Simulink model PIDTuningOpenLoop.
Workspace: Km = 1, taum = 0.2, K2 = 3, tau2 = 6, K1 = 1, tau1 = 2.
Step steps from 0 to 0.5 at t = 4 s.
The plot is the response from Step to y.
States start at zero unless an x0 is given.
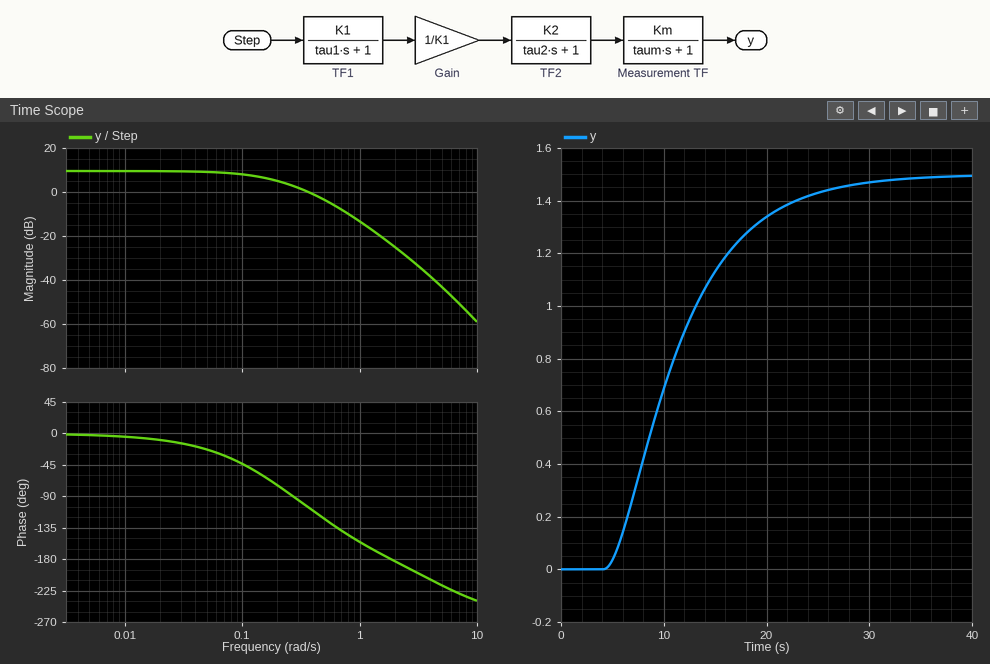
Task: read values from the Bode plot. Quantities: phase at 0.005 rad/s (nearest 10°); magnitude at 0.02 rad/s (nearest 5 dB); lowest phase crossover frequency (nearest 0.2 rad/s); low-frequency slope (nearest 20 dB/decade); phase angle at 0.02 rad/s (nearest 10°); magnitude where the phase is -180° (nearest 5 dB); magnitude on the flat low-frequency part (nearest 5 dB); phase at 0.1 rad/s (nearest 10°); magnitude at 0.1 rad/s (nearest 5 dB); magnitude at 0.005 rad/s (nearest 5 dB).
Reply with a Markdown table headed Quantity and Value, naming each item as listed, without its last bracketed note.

| Quantity | Value |
|---|---|
| phase at 0.005 rad/s | 0° |
| magnitude at 0.02 rad/s | 10 dB |
| lowest phase crossover frequency | 1.8 rad/s |
| low-frequency slope | 0 dB/decade |
| phase angle at 0.02 rad/s | -10° |
| magnitude where the phase is -180° | -25 dB |
| magnitude on the flat low-frequency part | 10 dB |
| phase at 0.1 rad/s | -40° |
| magnitude at 0.1 rad/s | 10 dB |
| magnitude at 0.005 rad/s | 10 dB |
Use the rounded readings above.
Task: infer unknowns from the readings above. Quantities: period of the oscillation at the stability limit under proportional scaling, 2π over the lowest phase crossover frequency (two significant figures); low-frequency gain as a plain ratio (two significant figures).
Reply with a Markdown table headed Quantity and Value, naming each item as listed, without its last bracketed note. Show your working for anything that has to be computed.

| Quantity | Value |
|---|---|
| period of the oscillation at the stability limit under proportional scaling, 2π over the lowest phase crossover frequency | 2π / 1.8 = 3.5 s |
| low-frequency gain as a plain ratio | 10^(10 / 20) = 3.2 |
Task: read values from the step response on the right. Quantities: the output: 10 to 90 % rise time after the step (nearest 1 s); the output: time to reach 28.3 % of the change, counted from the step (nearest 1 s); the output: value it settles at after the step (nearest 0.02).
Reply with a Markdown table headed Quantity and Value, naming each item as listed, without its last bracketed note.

| Quantity | Value |
|---|---|
| the output: 10 to 90 % rise time after the step | 14 s |
| the output: time to reach 28.3 % of the change, counted from the step | 4 s |
| the output: value it settles at after the step | 1.50 |
